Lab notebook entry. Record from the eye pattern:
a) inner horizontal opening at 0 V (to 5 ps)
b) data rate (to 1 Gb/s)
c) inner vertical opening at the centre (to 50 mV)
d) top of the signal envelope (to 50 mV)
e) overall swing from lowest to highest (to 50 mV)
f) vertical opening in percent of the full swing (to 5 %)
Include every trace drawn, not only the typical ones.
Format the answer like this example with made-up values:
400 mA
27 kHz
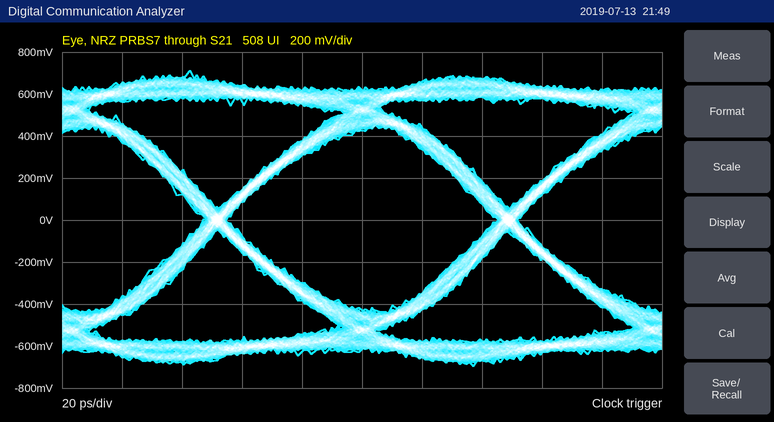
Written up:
90 ps
10 Gb/s
850 mV
700 mV
1.40 V
60 %
